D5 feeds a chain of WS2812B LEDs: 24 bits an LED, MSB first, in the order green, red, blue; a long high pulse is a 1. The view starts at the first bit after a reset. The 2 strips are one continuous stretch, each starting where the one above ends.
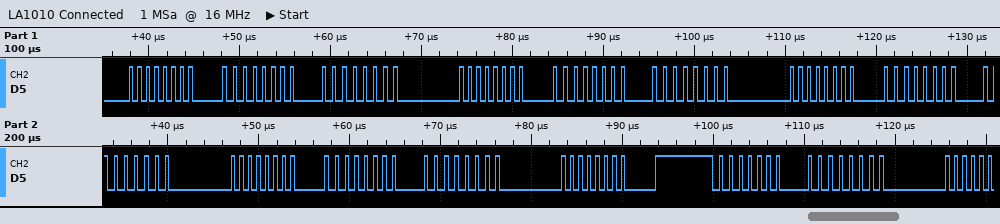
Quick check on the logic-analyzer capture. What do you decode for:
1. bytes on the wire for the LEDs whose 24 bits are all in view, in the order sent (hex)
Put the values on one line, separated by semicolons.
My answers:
00 00 00 00 00 00 00 00 00 00 00 00 00 80 00
